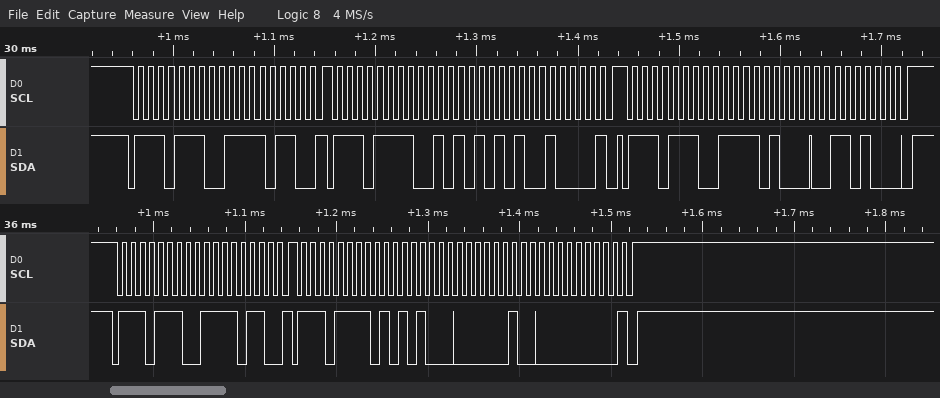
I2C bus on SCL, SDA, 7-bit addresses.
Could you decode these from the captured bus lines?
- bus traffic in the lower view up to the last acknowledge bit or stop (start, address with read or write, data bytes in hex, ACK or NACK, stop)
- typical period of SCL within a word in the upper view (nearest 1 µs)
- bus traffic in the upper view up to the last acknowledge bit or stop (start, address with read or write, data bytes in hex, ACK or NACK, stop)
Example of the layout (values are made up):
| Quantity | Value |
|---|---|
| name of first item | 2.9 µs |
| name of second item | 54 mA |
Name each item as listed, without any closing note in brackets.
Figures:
| Quantity | Value |
|---|---|
| bus traffic in the lower view up to the last acknowledge bit or stop | start, address 77 write ACK, F6 ACK, repeated start, address 77 read ACK, A8 ACK, 04 ACK, 00 NACK, stop |
| typical period of SCL within a word in the upper view | 10 µs |
| bus traffic in the upper view up to the last acknowledge bit or stop | start, address 77 write ACK, F6 ACK, repeated start, address 77 read ACK, 55 ACK, 90 NACK, stop, start, address 77 write ACK, F4 ACK, 34 ACK, stop |
